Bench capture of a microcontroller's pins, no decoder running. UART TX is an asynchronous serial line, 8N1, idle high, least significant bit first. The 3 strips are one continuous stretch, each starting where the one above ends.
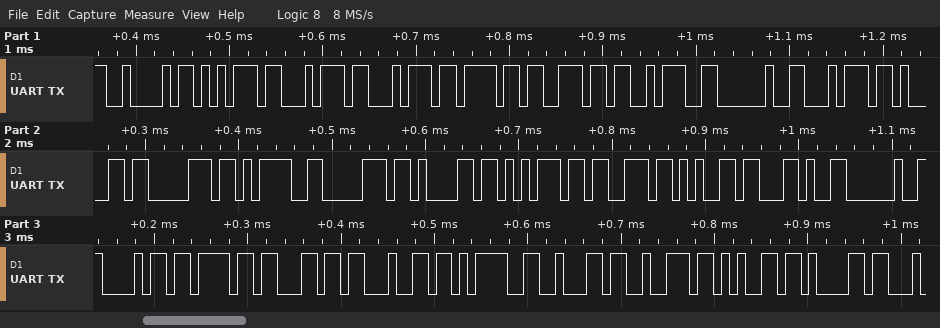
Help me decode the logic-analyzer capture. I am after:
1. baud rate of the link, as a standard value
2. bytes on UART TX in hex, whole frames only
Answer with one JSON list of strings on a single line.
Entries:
["115200 baud", "42 75 74 74 6F 6E 3A 20 74 61 70 3D 70 61 75 73 65 2C 20 68 6F 6C 64 3D 62 72 65 61"]
